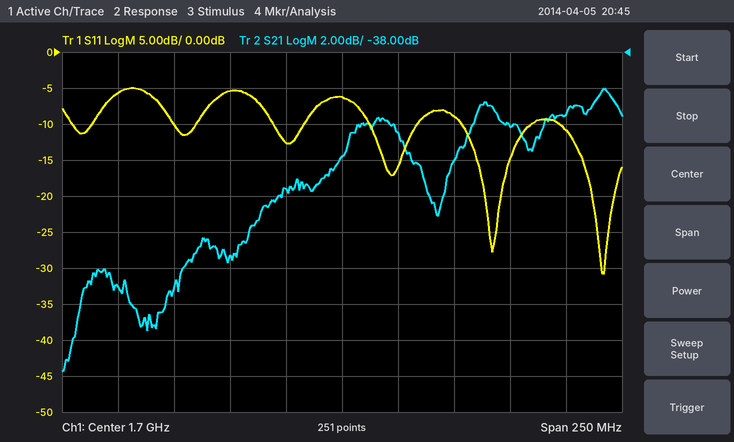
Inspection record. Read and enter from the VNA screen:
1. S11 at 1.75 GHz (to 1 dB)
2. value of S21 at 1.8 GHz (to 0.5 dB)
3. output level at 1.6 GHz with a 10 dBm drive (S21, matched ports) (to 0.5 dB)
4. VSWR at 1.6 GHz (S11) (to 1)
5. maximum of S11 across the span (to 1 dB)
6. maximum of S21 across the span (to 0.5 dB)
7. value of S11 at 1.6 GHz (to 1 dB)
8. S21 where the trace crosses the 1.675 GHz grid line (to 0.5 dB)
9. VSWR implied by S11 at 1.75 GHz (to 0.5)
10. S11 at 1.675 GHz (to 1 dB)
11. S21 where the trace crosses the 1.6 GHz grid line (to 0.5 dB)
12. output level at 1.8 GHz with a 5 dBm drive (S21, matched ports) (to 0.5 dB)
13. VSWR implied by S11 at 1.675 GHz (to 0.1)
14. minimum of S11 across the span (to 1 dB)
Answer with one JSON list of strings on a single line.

["-9 dB", "-41.5 dB", "-41.0 dBm", "3", "-5 dB", "-40.0 dB", "-6 dB", "-45.5 dB", "2.0", "-13 dB", "-51.0 dB", "-36.5 dBm", "1.6", "-31 dB"]
